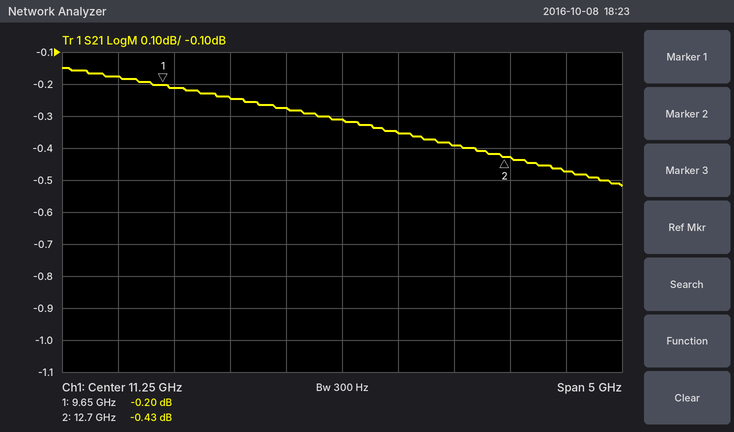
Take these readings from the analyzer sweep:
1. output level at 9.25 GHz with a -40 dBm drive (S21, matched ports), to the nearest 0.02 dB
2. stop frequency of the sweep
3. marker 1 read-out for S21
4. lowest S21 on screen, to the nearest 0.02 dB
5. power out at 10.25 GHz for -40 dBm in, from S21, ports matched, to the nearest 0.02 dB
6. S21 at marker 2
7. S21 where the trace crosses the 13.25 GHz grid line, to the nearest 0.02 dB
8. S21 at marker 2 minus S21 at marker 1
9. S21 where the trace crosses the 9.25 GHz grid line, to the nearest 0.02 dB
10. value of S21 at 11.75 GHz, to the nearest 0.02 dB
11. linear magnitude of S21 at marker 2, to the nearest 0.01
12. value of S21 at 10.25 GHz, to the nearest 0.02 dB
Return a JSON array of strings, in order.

["-40.18 dBm", "13.75 GHz", "-0.20 dB", "-0.52 dB", "-40.24 dBm", "-0.43 dB", "-0.48 dB", "-0.23 dB", "-0.18 dB", "-0.36 dB", "0.95", "-0.24 dB"]
